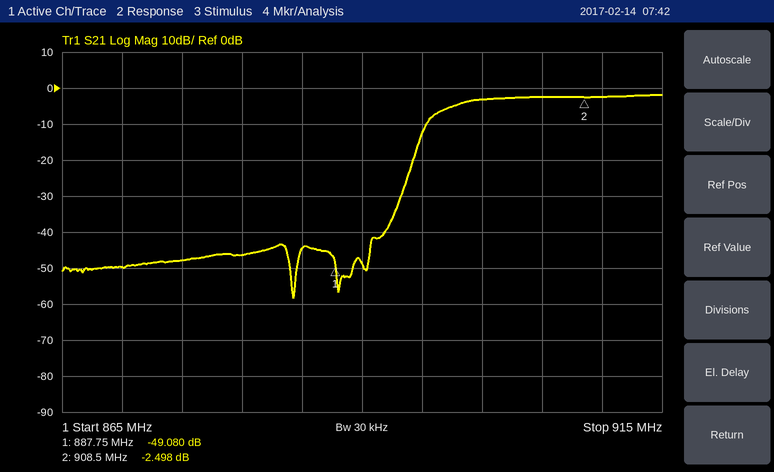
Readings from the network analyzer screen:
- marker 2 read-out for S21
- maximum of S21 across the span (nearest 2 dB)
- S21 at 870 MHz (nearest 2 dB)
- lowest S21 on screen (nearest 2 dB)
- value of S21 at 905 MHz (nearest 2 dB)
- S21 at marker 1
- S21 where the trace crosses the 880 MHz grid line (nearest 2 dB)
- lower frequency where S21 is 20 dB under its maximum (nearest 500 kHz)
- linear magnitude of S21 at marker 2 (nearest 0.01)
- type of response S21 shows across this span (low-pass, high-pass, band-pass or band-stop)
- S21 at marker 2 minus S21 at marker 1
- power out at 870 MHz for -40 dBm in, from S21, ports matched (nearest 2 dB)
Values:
-2.498 dB
-2 dB
-50 dB
-58 dB
-2 dB
-49.080 dB
-46 dB
894.0 MHz
0.75
high-pass
46.582 dB
-90 dBm
